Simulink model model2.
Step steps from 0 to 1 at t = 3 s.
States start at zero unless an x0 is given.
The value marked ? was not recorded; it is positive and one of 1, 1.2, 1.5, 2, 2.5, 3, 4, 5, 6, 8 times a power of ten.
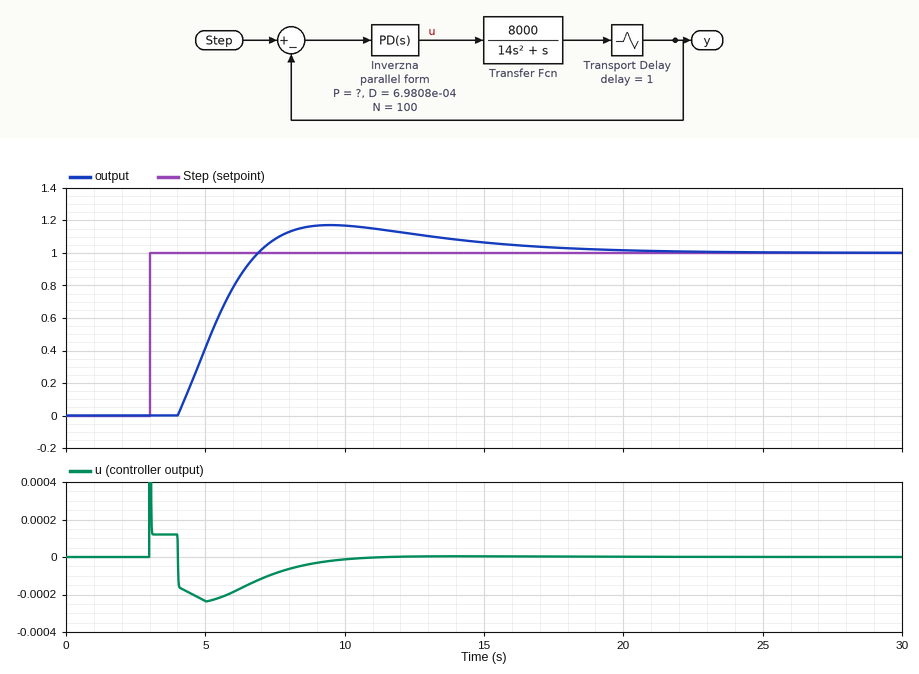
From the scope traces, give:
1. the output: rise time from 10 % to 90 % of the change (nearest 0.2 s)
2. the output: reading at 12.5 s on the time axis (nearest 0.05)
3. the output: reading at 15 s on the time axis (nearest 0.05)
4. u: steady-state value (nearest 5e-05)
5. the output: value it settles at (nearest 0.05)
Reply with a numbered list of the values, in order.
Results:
1. 2.2 s
2. 1.10
3. 1.05
4. 0.00000
5. 1.00
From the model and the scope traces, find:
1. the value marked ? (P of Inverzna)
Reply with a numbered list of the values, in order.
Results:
1. 0.00012
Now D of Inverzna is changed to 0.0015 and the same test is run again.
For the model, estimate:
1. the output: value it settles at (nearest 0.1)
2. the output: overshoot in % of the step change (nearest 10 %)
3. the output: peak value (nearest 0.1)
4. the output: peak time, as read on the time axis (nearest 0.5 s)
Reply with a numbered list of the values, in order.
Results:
1. 1.0
2. 40 %
3. 1.4
4. 6.0 s
